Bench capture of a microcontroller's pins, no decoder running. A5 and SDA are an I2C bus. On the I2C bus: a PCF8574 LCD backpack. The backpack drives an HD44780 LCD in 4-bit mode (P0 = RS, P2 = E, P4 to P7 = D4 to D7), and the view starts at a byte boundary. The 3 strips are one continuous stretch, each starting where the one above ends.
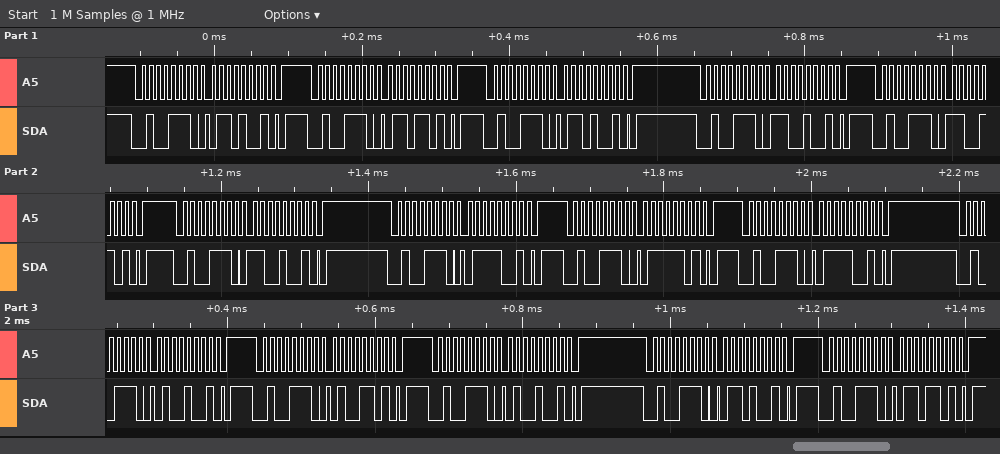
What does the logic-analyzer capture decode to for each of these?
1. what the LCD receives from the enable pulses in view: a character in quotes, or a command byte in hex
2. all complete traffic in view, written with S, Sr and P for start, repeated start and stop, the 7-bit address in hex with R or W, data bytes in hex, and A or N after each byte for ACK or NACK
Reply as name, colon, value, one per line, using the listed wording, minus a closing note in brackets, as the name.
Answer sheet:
what the LCD receives from the enable pulses in view: a character in quotes, or a command byte in hex: 'l' 't'
all complete traffic in view, written with S, Sr and P for start, repeated start and stop, the 7-bit address in hex with R or W, data bytes in hex, and A or N after each byte for ACK or NACK: S 27W A 69 A P S 27W A 6D A P S 27W A 69 A P S 27W A C9 A P S 27W A CD A P S 27W A C9 A P S 27W A 79 A P S 27W A 7D A P S 27W A 79 A P S 27W A 49 A P S 27W A 4D A P S 27W A 49 A P S 27W A 69 A P S 27W A 6D A P
